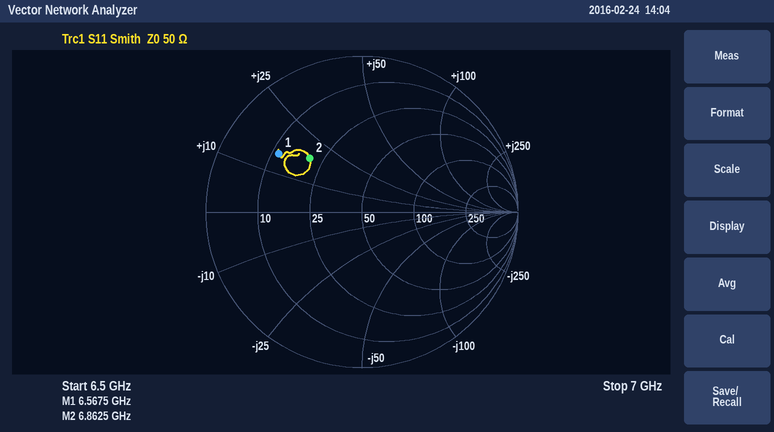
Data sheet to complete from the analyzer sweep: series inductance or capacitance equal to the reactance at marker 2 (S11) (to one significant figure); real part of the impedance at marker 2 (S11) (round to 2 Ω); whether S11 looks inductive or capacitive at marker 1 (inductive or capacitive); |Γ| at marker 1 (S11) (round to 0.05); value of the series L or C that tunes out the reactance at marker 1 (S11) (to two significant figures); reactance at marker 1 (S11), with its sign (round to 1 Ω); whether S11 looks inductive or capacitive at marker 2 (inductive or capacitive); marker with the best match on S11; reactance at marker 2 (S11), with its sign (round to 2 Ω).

400 pH
20 Ω
inductive
0.65
1.6 pF
+15 Ω
inductive
marker 2
+18 Ω
